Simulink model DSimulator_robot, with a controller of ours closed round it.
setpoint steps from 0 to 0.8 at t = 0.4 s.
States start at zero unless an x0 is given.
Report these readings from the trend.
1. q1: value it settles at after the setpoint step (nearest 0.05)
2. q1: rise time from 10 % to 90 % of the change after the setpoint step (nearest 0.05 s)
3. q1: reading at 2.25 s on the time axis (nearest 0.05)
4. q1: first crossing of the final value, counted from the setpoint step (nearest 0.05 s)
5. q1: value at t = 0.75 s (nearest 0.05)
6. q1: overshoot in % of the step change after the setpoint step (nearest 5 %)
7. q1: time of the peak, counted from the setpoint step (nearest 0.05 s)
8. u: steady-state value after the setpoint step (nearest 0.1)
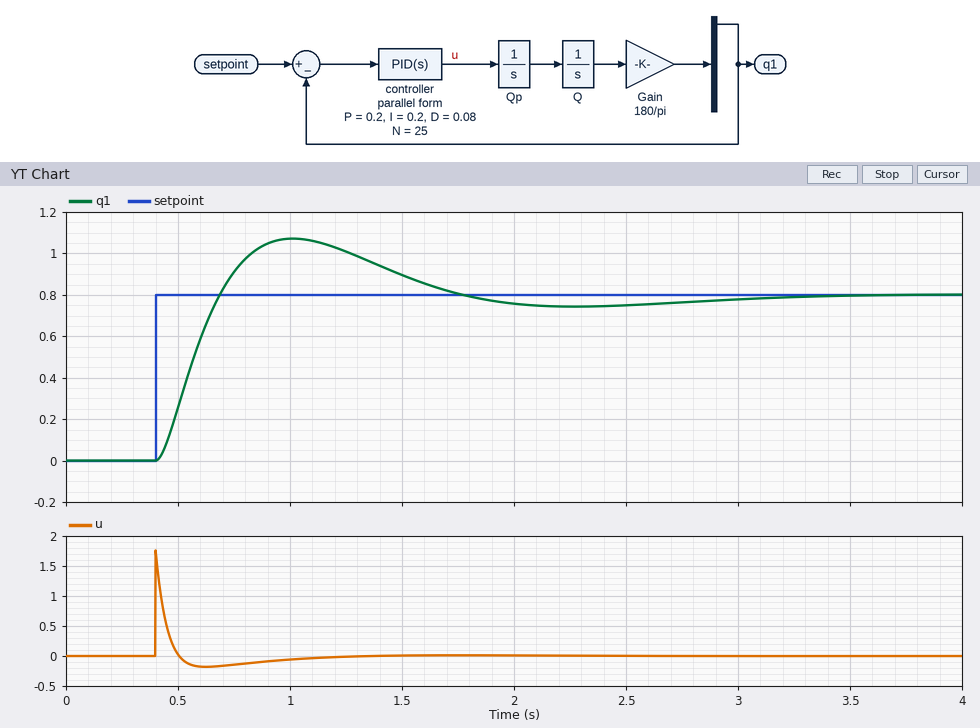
0.80
0.20 s
0.75
0.30 s
0.90
35 %
0.60 s
0.0
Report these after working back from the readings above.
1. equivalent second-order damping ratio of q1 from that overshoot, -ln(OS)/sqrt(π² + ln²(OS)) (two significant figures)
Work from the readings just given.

0.32
